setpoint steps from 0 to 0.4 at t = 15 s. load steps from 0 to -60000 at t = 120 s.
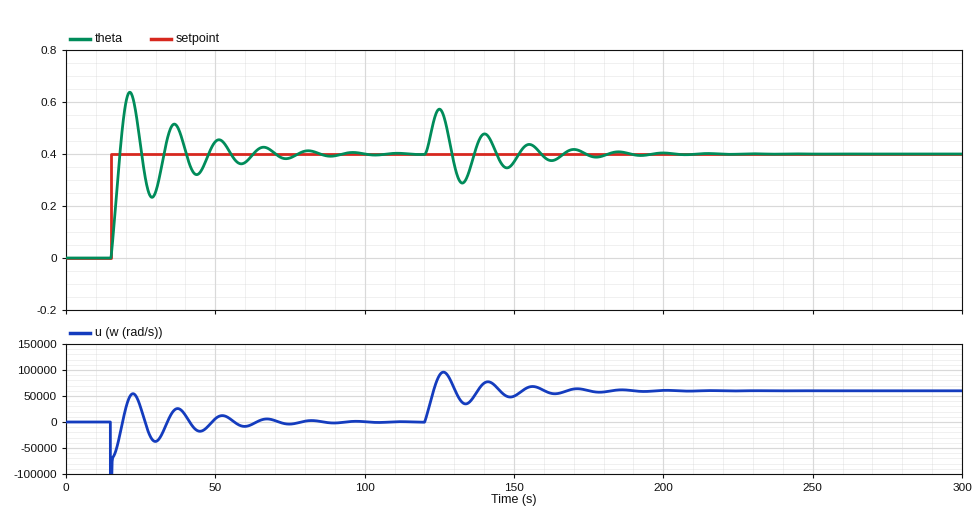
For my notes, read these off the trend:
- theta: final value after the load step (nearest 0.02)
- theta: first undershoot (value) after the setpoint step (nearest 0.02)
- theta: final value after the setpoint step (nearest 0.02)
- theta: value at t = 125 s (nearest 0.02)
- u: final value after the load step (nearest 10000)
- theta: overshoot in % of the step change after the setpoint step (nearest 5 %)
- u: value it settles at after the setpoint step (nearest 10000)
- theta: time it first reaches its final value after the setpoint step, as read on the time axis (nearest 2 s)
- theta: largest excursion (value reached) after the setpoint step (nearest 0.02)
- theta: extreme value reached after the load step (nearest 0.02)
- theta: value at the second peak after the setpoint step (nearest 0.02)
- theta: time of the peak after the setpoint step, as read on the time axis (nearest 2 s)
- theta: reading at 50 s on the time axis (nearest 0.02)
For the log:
0.40
0.24
0.40
0.58
60000
60 %
0
18 s
0.64
0.58
0.52
22 s
0.44
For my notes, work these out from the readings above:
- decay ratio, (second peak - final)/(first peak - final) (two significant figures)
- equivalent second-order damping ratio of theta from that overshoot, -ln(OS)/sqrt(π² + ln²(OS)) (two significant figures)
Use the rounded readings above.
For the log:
0.50
0.16
